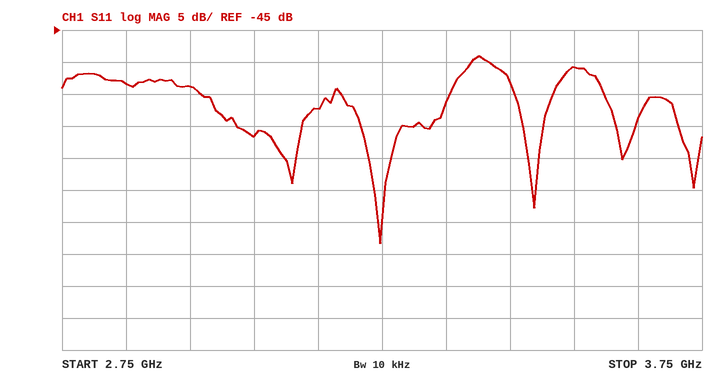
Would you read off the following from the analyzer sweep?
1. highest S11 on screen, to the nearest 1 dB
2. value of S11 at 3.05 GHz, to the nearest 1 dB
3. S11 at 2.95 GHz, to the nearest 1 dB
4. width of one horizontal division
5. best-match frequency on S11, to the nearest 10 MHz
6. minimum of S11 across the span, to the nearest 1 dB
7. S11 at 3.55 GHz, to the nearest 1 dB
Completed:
-49 dB
-62 dB
-54 dB
100 MHz
3.25 GHz
-78 dB
-51 dB
